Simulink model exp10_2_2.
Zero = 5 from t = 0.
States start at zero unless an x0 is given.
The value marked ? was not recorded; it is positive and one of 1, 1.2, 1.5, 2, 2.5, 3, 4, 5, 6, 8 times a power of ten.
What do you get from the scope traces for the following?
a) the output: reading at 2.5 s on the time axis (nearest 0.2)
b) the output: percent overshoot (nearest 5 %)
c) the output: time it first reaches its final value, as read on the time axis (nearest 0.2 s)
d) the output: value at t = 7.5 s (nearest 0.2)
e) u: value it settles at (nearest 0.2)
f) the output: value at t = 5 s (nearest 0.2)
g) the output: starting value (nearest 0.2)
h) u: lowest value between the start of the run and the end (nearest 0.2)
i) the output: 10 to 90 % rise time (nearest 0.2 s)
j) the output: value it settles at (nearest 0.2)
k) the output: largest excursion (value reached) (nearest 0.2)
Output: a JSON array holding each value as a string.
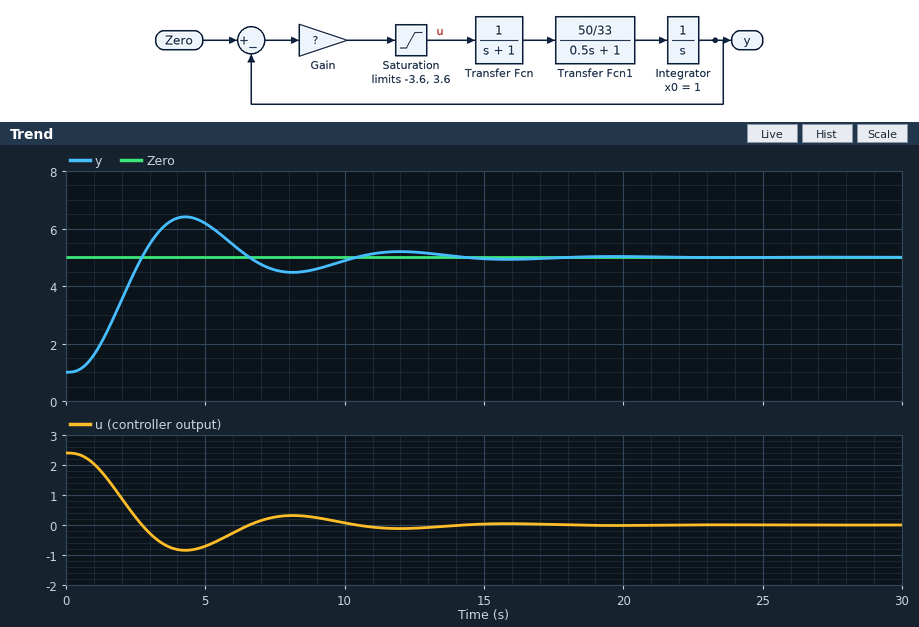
["4.6", "35 %", "2.8 s", "4.6", "0.0", "6.2", "1.0", "-0.8", "1.6 s", "5.0", "6.4"]
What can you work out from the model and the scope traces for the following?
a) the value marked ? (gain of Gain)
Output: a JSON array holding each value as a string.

["0.6"]
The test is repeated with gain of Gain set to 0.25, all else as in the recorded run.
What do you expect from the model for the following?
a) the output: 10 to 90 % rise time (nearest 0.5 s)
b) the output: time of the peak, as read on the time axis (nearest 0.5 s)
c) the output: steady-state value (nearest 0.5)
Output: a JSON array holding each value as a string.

["3.5 s", "7.5 s", "5.0"]
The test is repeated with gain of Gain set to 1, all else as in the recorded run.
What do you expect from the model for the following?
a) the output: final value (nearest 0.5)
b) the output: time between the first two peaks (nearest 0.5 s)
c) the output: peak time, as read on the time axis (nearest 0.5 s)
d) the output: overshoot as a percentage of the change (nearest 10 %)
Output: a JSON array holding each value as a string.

["5.0", "6.0 s", "3.5 s", "60 %"]
